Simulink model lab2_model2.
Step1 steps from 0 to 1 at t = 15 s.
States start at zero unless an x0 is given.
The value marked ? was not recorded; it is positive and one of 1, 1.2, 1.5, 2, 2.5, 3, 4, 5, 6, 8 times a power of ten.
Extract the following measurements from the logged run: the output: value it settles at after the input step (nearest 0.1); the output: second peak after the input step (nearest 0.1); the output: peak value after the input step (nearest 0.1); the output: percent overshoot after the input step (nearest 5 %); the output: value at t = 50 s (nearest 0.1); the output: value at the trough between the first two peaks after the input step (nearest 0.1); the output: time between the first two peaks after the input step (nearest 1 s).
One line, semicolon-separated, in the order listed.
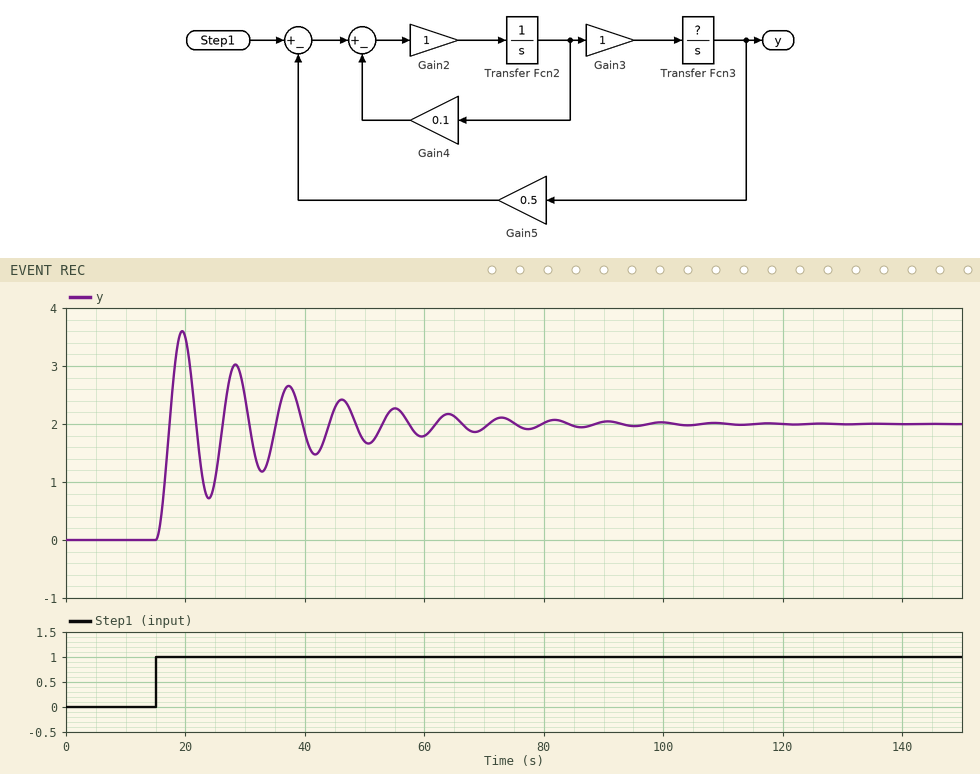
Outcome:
2.0; 3.0; 3.6; 80 %; 1.7; 0.7; 9 s
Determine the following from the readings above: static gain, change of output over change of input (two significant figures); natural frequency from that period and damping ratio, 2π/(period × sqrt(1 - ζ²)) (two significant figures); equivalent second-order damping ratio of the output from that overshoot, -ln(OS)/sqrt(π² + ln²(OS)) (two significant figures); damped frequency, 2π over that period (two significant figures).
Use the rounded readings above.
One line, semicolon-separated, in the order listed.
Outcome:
2.0; 0.70 rad/s; 0.071; 0.70 rad/s
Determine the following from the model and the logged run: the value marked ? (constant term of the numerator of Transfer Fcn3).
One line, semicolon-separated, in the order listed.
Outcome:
1
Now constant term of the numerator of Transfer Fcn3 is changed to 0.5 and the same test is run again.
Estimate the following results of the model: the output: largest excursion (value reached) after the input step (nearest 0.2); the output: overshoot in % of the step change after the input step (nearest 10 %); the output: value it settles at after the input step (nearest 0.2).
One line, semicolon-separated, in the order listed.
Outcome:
3.4; 70 %; 2.0
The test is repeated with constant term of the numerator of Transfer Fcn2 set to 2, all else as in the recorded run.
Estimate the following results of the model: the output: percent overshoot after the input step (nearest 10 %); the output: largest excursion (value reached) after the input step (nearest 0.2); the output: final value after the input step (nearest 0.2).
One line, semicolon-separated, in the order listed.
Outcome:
70 %; 3.4; 2.0
